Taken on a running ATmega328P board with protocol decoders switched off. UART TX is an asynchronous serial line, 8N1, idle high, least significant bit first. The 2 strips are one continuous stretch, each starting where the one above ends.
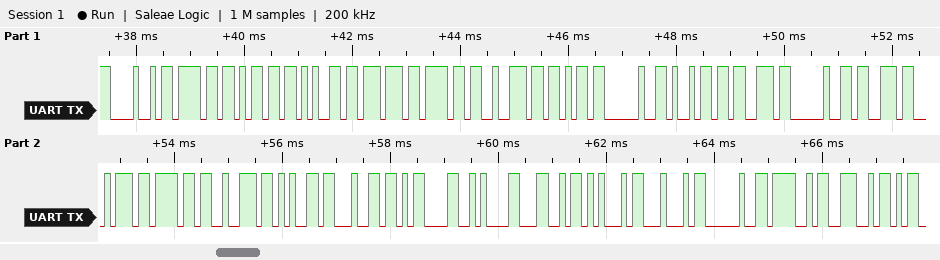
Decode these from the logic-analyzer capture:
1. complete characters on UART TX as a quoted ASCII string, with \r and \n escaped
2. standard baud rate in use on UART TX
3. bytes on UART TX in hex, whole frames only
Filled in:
"Homework is stored\r\nLED ON"
9600 baud
0x48 0x6F 0x6D 0x65 0x77 0x6F 0x72 0x6B 0x20 0x69 0x73 0x20 0x73 0x74 0x6F 0x72 0x65 0x64 0x0D 0x0A 0x4C 0x45 0x44 0x20 0x4F 0x4E
